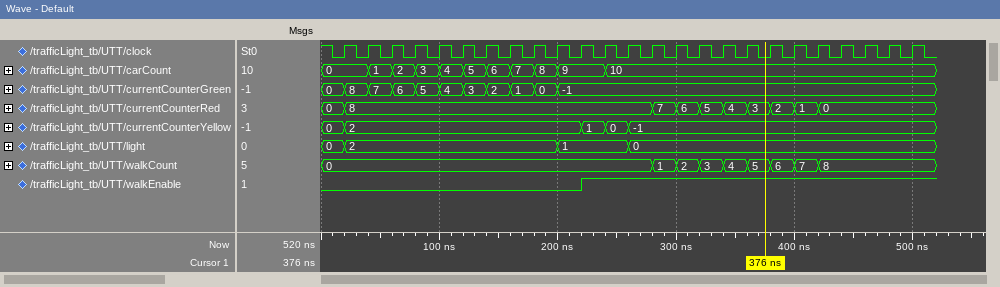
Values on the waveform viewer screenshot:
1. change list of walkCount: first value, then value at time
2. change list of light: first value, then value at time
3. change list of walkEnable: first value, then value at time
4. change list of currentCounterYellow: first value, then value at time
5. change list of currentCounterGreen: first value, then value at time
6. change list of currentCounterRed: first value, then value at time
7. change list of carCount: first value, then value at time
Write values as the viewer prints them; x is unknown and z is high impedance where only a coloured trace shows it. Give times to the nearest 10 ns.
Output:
0, 1 at 280 ns, 2 at 300 ns, 3 at 320 ns, 4 at 340 ns, 5 at 360 ns, 6 at 380 ns, 7 at 400 ns, 8 at 420 ns
0, 2 at 20 ns, 1 at 200 ns, 0 at 260 ns
0, 1 at 220 ns
0, 2 at 20 ns, 1 at 220 ns, 0 at 240 ns, -1 at 260 ns
0, 8 at 20 ns, 7 at 40 ns, 6 at 60 ns, 5 at 80 ns, 4 at 100 ns, 3 at 120 ns, 2 at 140 ns, 1 at 160 ns, 0 at 180 ns, -1 at 200 ns
0, 8 at 20 ns, 7 at 280 ns, 6 at 300 ns, 5 at 320 ns, 4 at 340 ns, 3 at 360 ns, 2 at 380 ns, 1 at 400 ns, 0 at 420 ns
0, 1 at 40 ns, 2 at 60 ns, 3 at 80 ns, 4 at 100 ns, 5 at 120 ns, 6 at 140 ns, 7 at 160 ns, 8 at 180 ns, 9 at 200 ns, 10 at 240 ns
